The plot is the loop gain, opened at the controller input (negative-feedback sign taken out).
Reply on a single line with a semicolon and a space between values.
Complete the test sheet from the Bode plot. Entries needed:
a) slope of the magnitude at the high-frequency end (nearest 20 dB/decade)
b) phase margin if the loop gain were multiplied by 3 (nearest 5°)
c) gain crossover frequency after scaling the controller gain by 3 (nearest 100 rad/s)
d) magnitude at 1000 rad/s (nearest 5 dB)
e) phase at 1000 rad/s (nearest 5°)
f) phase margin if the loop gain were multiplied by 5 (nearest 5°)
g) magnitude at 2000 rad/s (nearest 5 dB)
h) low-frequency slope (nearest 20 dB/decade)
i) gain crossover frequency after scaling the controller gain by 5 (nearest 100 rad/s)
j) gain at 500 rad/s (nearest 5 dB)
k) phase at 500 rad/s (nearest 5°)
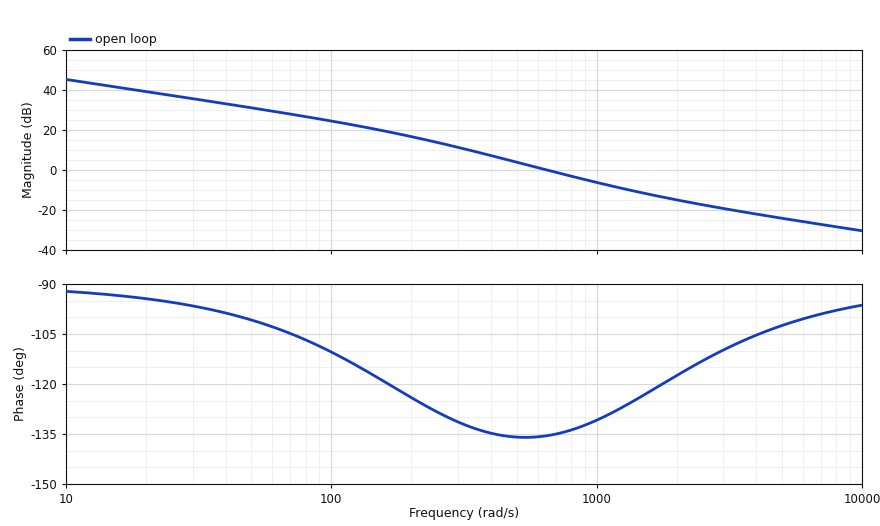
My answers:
-20 dB/decade; 55°; 1300 rad/s; -5 dB; -130°; 60°; -15 dB; -20 dB/decade; 1800 rad/s; 5 dB; -135°
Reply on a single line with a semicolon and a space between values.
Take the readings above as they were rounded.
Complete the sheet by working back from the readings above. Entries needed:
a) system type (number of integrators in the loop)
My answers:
1
